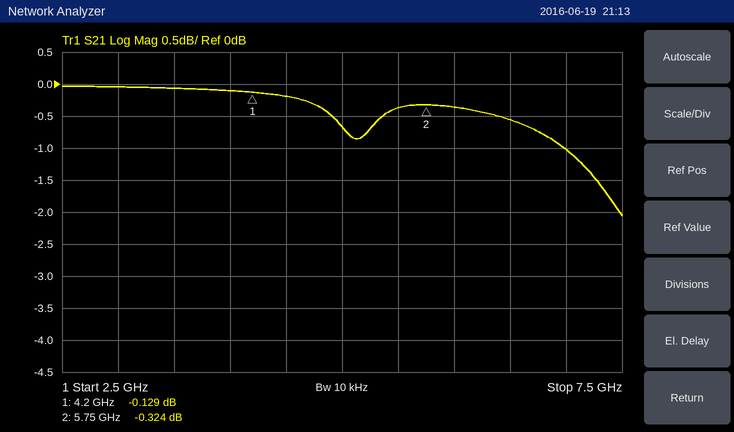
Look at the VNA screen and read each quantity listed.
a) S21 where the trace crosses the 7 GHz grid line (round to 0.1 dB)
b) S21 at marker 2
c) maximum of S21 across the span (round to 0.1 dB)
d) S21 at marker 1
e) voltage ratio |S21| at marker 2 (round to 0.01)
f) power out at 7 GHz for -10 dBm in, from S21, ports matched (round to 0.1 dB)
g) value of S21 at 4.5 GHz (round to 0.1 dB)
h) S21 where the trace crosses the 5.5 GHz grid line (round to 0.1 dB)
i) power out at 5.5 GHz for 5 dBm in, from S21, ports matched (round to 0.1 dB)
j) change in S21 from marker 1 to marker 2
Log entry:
-1.0 dB
-0.324 dB
0.0 dB
-0.129 dB
0.96
-11.0 dBm
-0.2 dB
-0.4 dB
4.6 dBm
-0.195 dB
